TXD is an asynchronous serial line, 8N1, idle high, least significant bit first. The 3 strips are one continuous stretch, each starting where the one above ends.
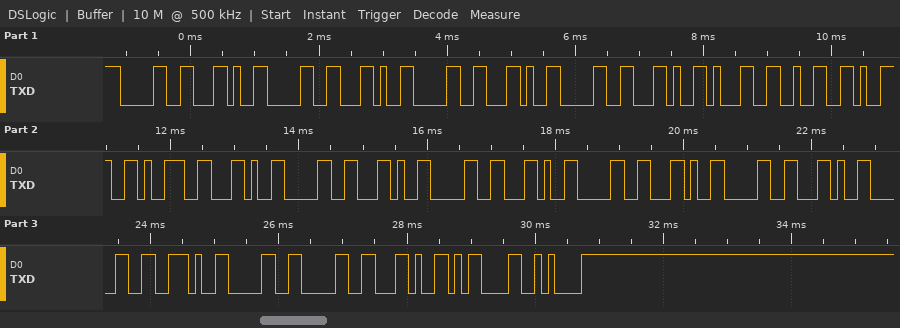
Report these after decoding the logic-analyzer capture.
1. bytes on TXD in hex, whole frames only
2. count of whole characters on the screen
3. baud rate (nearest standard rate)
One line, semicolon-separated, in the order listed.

30 2C 30 2C 30 2C 30 2C 31 32 39 39 2C 30 2C 30 2C 30 2C 30 2C 30 2E 30 30 2C 0D 0A; 28; 9600 baud
